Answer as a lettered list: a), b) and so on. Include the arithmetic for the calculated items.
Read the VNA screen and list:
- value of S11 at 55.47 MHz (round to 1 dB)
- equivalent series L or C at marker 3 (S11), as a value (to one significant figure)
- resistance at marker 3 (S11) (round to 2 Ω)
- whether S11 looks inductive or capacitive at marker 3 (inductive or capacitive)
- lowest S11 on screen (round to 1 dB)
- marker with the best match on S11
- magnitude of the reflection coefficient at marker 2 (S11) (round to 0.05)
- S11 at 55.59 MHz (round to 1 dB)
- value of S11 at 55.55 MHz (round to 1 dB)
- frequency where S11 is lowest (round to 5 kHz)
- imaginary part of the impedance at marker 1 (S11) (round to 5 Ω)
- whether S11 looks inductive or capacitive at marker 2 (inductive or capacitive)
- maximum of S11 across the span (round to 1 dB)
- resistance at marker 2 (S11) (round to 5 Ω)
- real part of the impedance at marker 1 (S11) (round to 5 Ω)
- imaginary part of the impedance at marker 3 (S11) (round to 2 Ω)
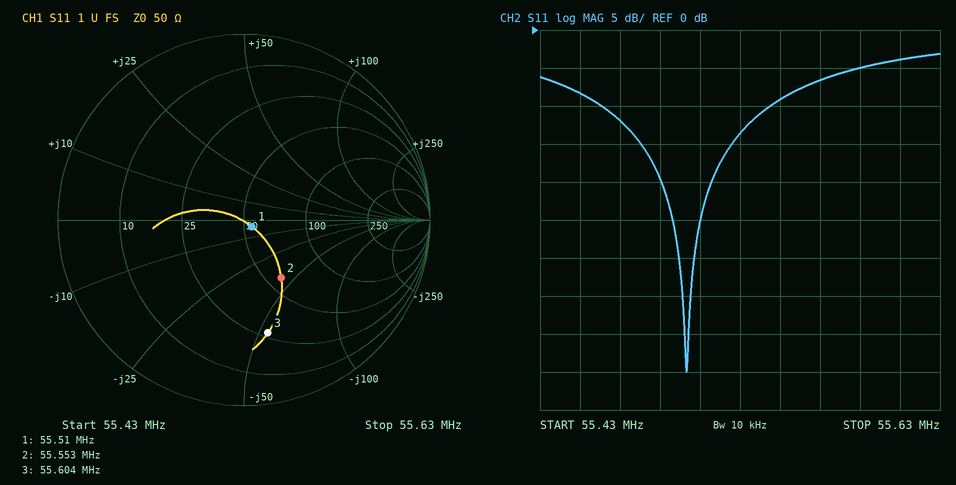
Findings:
a) -12 dB
b) C = 1/(2π × 55.604 MHz × 54 Ω) ≈ 53.0 pF, so 50 pF to one significant figure
c) 28 Ω
d) capacitive
e) -45 dB
f) marker 1
g) 0.35
h) -5 dB
i) -9 dB
j) 55.505 MHz
k) -5 Ω
l) capacitive
m) -3 dB
n) 60 Ω
o) 55 Ω
p) -54 Ω
